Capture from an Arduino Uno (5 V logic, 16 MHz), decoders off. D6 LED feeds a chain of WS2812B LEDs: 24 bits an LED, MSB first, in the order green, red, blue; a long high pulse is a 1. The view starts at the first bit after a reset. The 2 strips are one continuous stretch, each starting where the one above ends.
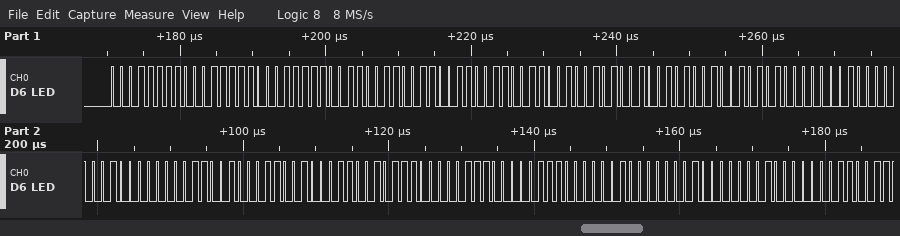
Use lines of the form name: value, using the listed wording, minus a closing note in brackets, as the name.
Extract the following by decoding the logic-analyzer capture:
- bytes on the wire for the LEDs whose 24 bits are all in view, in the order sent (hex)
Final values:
bytes on the wire for the LEDs whose 24 bits are all in view, in the order sent: 1F 1F 1F 33 33 33 25 25 25 40 40 40 32 32 32 E0 E0 E0 40 40 40
